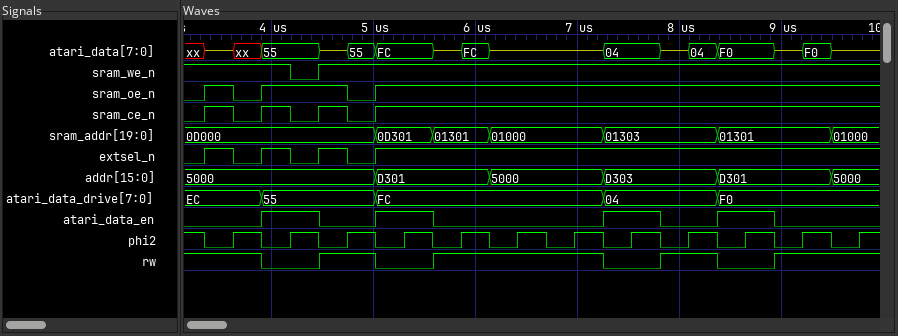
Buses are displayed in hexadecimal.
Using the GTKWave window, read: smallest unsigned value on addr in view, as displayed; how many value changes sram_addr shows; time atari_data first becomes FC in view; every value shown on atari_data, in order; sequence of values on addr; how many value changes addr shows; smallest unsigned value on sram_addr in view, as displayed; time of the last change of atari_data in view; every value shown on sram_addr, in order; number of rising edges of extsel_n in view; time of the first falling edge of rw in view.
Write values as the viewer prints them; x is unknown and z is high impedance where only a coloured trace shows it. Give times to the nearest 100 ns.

5000
6
5000 ns
xx, z, xx, 55, z, 55, FC, z, FC, z, 04, z, 04, F0, z, F0, z
5000, D301, 5000, D303, D301, 5000
5
01000
9500 ns
0D000, 0D301, 01301, 01000, 01303, 01301, 01000
4
3900 ns
